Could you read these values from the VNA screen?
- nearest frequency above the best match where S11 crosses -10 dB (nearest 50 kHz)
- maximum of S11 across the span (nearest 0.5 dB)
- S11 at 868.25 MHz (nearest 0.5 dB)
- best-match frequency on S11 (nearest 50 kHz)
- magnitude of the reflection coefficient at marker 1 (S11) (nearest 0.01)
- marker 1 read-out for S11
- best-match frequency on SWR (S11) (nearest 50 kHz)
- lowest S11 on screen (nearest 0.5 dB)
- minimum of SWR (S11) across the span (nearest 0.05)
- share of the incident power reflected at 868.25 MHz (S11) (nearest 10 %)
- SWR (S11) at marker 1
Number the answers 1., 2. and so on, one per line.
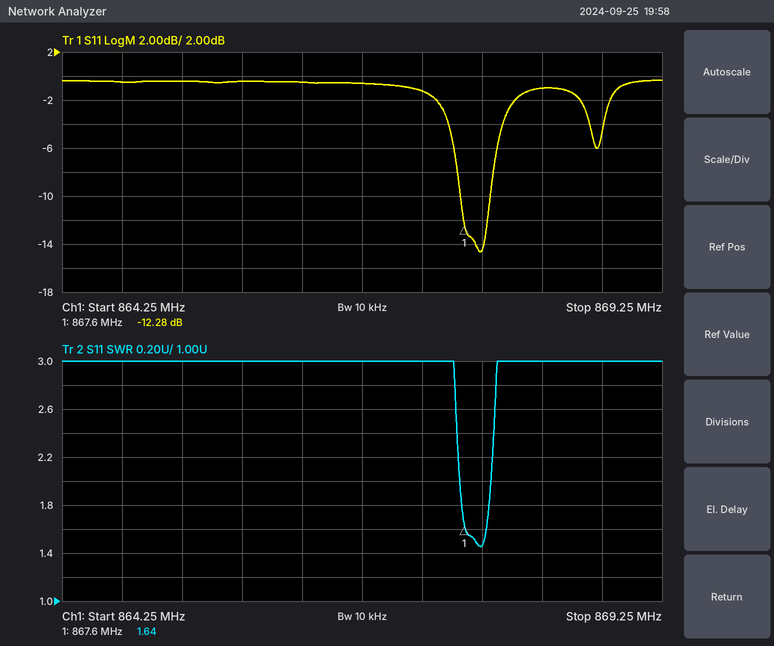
1. 867.80 MHz
2. -0.5 dB
3. -1.0 dB
4. 867.75 MHz
5. 0.24
6. -12.28 dB
7. 867.75 MHz
8. -14.5 dB
9. 1.45
10. 80 %
11. 1.64
